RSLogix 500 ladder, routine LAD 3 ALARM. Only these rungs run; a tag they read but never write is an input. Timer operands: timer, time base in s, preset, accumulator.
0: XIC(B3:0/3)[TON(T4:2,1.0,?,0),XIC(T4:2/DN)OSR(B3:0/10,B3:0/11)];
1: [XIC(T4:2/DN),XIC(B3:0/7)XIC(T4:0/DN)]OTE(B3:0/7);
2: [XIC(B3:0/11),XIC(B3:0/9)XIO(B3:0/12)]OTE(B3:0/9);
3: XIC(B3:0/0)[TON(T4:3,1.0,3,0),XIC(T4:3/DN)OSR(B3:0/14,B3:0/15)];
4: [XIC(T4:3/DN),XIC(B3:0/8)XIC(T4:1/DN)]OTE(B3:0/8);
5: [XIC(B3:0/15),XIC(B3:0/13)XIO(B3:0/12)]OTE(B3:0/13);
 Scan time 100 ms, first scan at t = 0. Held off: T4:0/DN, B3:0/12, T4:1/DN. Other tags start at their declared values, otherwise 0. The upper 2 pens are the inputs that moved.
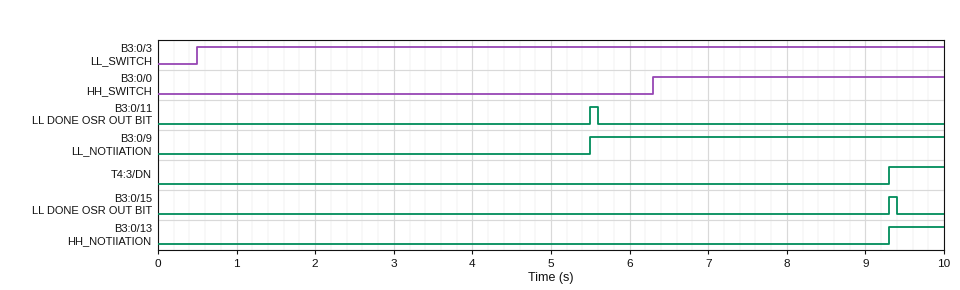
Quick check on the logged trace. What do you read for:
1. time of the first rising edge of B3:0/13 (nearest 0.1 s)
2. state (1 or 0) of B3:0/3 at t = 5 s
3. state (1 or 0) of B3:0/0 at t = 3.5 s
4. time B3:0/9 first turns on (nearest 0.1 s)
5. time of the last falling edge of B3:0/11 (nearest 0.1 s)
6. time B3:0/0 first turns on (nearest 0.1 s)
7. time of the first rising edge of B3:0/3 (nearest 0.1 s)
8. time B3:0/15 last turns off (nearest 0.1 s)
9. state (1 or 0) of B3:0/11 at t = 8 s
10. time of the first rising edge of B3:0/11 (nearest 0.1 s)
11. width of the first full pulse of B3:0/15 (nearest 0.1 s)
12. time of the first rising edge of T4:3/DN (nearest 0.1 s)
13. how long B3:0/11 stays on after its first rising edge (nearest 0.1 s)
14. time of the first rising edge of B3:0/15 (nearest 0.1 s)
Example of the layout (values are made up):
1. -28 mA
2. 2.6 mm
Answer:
1. 9.3 s
2. 1
3. 0
4. 5.5 s
5. 5.6 s
6. 6.3 s
7. 0.5 s
8. 9.4 s
9. 0
10. 5.5 s
11. 0.1 s
12. 9.3 s
13. 0.1 s
14. 9.3 s
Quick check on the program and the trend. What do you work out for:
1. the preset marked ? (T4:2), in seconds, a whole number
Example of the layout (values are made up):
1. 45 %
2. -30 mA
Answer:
1. 5 s
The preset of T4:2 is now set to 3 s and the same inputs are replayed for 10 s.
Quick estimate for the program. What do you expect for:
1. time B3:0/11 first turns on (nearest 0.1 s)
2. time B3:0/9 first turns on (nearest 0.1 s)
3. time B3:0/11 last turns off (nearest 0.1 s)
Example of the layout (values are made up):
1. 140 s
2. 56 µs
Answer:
1. 3.5 s
2. 3.5 s
3. 3.6 s
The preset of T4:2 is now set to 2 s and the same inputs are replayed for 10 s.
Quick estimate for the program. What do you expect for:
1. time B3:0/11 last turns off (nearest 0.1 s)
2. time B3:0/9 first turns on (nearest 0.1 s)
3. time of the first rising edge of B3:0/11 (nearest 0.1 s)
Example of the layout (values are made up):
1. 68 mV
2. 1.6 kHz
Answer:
1. 2.6 s
2. 2.5 s
3. 2.5 s
